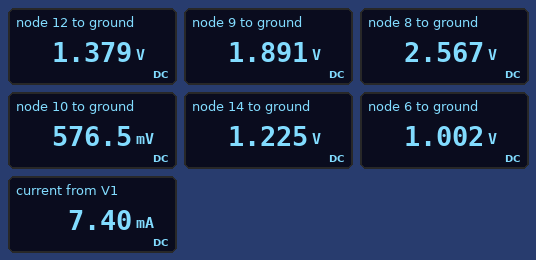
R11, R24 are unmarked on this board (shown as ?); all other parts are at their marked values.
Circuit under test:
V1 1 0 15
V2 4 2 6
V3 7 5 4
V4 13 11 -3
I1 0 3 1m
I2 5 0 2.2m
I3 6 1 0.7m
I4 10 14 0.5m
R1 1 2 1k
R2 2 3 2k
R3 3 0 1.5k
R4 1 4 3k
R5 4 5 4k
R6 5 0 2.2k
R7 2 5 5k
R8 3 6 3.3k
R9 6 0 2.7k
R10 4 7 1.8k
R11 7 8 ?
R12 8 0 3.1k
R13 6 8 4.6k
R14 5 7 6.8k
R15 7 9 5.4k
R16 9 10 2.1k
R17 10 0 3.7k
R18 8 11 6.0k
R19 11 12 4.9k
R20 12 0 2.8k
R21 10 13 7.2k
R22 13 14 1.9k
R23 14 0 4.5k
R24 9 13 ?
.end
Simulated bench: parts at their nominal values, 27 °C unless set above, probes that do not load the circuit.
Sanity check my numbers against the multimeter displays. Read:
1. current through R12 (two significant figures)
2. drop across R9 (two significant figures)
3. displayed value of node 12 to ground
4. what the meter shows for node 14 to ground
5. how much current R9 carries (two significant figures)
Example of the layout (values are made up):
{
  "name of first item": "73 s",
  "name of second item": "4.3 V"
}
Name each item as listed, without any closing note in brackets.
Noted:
{
  "current through R12": "830 µA",
  "drop across R9": "1.0 V",
  "displayed value of node 12 to ground": "1.379 V",
  "what the meter shows for node 14 to ground": "1.225 V",
  "how much current R9 carries": "370 µA"
}
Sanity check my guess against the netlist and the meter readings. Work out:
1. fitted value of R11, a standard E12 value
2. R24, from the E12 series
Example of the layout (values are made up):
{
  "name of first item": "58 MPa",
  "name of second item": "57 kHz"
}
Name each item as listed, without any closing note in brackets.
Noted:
{
  "fitted value of R11, a standard E12 value": "5.6 kΩ",
  "R24, from the E12 series": "2.2 kΩ"
}
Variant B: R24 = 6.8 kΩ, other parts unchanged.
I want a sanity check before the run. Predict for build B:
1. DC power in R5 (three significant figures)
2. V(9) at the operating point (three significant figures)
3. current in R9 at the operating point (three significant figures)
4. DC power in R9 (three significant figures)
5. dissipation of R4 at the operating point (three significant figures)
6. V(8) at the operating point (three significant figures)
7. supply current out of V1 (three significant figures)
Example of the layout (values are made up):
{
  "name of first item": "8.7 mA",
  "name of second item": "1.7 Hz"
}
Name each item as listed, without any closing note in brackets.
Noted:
{
  "DC power in R5": "22.2 mW",
  "V(9) at the operating point": "2.39 V",
  "current in R9 at the operating point": "367 µA",
  "DC power in R9": "363 µW",
  "dissipation of R4 at the operating point": "803 µW",
  "V(8) at the operating point": "2.51 V",
  "supply current out of V1": "7.37 mA"
}
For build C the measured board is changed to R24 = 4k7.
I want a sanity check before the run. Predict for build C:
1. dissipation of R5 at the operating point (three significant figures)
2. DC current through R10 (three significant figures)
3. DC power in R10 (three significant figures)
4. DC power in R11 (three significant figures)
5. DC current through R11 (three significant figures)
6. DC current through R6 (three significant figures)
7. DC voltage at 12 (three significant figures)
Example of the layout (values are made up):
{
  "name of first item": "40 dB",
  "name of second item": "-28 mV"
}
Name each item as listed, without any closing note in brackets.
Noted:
{
  "dissipation of R5 at the operating point": "22.3 mW",
  "DC current through R10": "3.02 mA",
  "DC power in R10": "16.4 mW",
  "DC power in R11": "5.35 mW",
  "DC current through R11": "977 µA",
  "DC current through R6": "1.82 mA",
  "DC voltage at 12": "1.30 V"
}
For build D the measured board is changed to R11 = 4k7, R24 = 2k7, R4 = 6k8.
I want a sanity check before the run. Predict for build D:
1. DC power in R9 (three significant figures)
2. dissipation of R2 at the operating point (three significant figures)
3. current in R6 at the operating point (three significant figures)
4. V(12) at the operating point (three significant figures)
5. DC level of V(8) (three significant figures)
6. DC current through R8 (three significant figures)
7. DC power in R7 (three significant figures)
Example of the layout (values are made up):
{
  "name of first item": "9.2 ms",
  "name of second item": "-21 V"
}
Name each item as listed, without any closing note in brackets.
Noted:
{
  "DC power in R9": "384 µW",
  "dissipation of R2 at the operating point": "7.54 mW",
  "current in R6 at the operating point": "1.72 mA",
  "V(12) at the operating point": "1.36 V",
  "DC level of V(8)": "2.72 V",
  "DC current through R8": "707 µA",
  "DC power in R7": "2.38 mW"
}
